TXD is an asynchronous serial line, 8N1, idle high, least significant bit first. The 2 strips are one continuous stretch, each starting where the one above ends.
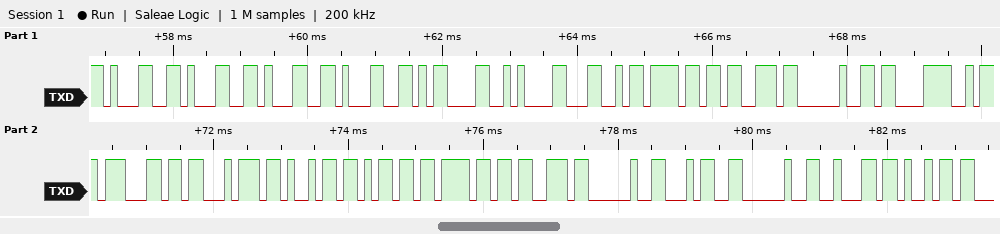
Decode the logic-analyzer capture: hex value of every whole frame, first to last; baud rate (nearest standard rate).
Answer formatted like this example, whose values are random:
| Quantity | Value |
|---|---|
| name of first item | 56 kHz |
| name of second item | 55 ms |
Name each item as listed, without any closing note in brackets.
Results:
| Quantity | Value |
|---|---|
| hex value of every whole frame, first to last | 0x31 0x31 0x31 0x31 0x0D 0x0A 0x4C 0x6F 0x73 0x20 0xC3 0xBA 0x6C 0x74 0x69 0x6D 0x6F 0x73 0x20 0x34 0x20 0x62 0x69 |
| baud rate | 9600 baud |
